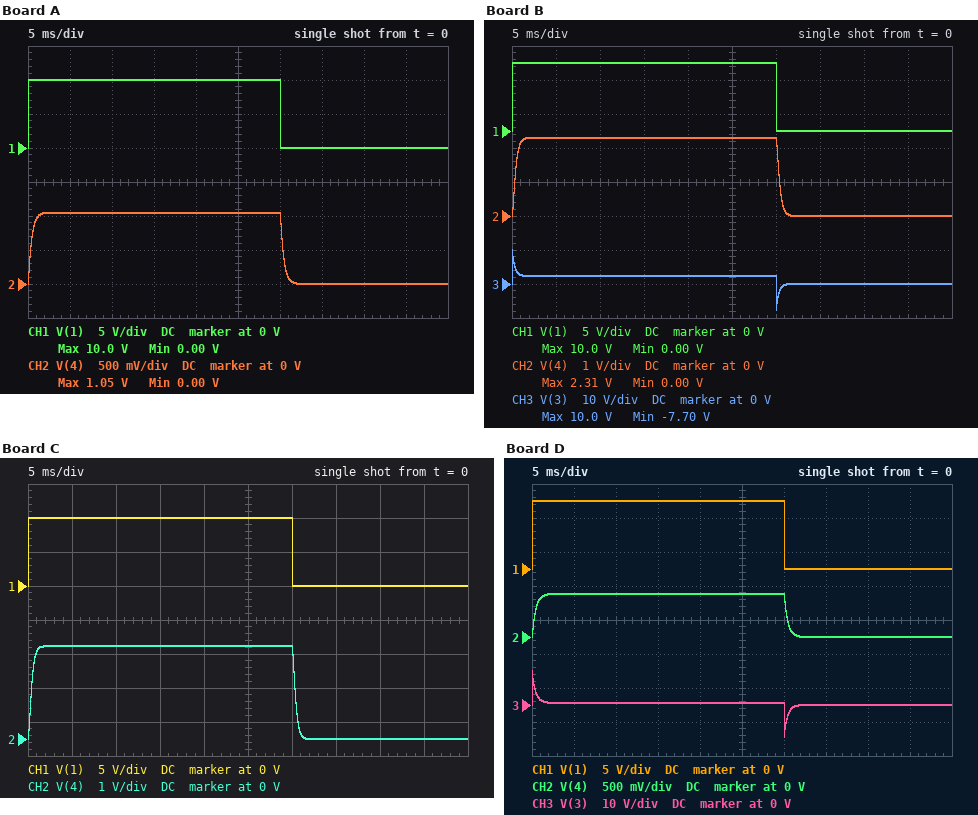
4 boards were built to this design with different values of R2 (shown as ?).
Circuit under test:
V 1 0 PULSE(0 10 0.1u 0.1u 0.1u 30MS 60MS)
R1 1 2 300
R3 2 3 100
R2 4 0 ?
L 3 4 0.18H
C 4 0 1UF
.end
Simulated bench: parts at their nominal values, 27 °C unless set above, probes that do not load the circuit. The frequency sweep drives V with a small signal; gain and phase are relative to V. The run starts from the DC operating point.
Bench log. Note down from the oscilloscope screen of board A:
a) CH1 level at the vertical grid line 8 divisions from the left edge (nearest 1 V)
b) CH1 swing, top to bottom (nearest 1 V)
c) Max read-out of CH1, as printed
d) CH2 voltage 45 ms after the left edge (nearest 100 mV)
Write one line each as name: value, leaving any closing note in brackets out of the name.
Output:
CH1 level at the vertical grid line 8 divisions from the left edge: 0 V
CH1 swing, top to bottom: 10 V
Max read-out of CH1, as printed: 10.0 V
CH2 voltage 45 ms after the left edge: 0 V
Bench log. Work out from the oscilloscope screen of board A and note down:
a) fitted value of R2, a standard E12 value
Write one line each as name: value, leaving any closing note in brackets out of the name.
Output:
fitted value of R2, a standard E12 value: 47 Ω
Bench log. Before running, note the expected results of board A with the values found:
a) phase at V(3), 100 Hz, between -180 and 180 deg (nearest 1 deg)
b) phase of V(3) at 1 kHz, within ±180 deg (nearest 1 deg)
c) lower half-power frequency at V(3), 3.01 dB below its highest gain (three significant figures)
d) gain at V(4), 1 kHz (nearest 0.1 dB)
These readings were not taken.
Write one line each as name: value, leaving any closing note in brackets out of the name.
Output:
phase at V(3), 100 Hz, between -180 and 180 deg: 53 deg
phase of V(3) at 1 kHz, within ±180 deg: 19 deg
lower half-power frequency at V(3), 3.01 dB below its highest gain: 395 Hz
gain at V(4), 1 kHz: -28.5 dB
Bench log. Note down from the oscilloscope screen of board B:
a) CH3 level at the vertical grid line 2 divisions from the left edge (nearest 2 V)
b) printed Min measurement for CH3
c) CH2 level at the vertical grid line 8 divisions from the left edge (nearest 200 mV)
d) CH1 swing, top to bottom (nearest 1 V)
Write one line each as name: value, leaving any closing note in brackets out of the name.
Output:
CH3 level at the vertical grid line 2 divisions from the left edge: 2 V
printed Min measurement for CH3: -7.70 V
CH2 level at the vertical grid line 8 divisions from the left edge: 0 V
CH1 swing, top to bottom: 10 V
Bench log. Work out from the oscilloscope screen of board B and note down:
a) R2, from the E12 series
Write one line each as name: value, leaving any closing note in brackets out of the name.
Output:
R2, from the E12 series: 120 Ω
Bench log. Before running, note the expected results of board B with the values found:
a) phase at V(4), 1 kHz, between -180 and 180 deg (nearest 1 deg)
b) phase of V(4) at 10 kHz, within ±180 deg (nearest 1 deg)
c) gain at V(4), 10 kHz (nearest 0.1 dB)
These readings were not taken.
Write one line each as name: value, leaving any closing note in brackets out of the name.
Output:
phase at V(4), 1 kHz, between -180 and 180 deg: -103 deg
phase of V(4) at 10 kHz, within ±180 deg: -170 deg
gain at V(4), 10 kHz: -57.1 dB
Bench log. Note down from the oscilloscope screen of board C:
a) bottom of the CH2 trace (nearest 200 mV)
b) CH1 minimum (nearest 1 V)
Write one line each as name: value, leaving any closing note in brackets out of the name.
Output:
bottom of the CH2 trace: 0 V
CH1 minimum: 0 V
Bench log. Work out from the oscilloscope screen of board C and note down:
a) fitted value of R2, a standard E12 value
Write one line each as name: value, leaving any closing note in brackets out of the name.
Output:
fitted value of R2, a standard E12 value: 150 Ω
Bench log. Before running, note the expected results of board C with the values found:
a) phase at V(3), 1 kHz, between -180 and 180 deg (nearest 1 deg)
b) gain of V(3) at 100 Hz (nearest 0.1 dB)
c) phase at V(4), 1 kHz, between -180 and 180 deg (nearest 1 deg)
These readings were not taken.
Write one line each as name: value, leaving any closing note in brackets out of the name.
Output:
phase at V(3), 1 kHz, between -180 and 180 deg: 20 deg
gain of V(3) at 100 Hz: -9.9 dB
phase at V(4), 1 kHz, between -180 and 180 deg: -109 deg
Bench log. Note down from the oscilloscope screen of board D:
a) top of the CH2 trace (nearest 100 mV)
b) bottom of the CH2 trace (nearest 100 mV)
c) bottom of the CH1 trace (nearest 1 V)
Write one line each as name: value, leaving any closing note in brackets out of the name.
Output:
top of the CH2 trace: 600 mV
bottom of the CH2 trace: 0 V
bottom of the CH1 trace: 0 V
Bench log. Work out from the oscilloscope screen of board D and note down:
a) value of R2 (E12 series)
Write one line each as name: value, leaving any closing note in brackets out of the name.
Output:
value of R2: 27 Ω
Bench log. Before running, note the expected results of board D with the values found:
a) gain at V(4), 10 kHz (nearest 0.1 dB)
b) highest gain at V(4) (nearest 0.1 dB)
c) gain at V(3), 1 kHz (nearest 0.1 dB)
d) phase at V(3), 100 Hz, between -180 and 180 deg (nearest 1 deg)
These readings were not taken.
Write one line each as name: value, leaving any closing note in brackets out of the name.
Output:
gain at V(4), 10 kHz: -58.3 dB
highest gain at V(4): -24.0 dB
gain at V(3), 1 kHz: -0.6 dB
phase at V(3), 100 Hz, between -180 and 180 deg: 62 deg
